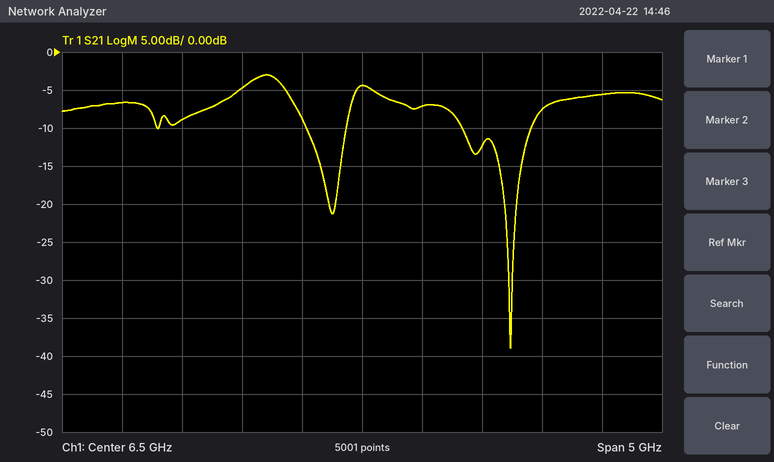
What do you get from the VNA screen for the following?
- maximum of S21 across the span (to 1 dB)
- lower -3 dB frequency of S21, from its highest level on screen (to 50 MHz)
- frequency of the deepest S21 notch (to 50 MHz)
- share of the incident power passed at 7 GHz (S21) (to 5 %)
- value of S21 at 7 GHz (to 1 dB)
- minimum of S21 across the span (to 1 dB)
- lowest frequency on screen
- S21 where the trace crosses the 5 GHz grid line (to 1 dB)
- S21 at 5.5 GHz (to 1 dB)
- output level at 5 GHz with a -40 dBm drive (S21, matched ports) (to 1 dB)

-3 dB
5.40 GHz
7.75 GHz
20 %
-7 dB
-39 dB
4 GHz
-9 dB
-5 dB
-49 dBm
